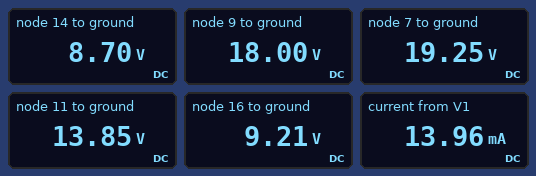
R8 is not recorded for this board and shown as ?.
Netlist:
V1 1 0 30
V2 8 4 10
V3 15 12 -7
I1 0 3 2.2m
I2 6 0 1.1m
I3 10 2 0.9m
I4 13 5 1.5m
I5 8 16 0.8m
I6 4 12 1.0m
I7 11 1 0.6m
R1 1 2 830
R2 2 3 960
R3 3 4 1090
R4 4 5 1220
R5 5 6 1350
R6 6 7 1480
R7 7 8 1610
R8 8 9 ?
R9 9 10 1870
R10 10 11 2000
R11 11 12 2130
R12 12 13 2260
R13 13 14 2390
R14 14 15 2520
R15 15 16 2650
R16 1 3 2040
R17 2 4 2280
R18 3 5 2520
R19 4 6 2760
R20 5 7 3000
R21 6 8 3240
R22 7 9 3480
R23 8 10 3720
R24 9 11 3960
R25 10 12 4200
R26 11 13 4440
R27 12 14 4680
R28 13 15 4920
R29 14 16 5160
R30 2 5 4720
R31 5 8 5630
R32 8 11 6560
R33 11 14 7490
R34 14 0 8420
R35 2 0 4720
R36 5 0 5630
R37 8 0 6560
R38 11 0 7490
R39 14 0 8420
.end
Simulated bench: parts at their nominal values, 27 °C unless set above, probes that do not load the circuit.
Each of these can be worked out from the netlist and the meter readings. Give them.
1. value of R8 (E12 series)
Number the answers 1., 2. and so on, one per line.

1. 3.3 kΩ
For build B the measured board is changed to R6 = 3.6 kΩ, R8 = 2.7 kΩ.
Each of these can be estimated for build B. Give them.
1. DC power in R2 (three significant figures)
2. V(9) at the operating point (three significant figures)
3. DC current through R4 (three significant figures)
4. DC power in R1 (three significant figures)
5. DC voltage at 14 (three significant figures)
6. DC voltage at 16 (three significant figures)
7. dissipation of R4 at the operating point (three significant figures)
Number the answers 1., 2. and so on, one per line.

1. 1.76 mW
2. 18.4 V
3. 3.12 mA
4. 81.7 mW
5. 8.85 V
6. 9.38 V
7. 11.9 mW
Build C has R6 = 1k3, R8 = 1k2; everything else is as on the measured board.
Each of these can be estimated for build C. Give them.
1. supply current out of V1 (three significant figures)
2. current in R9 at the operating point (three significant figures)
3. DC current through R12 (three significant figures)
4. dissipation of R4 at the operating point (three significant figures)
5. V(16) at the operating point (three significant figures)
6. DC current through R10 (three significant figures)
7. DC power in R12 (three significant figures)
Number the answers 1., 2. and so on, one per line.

1. 14.1 mA
2. 1.28 mA
3. 1.86 mA
4. 13.0 mW
5. 9.82 V
6. 1.35 mA
7. 7.83 mW
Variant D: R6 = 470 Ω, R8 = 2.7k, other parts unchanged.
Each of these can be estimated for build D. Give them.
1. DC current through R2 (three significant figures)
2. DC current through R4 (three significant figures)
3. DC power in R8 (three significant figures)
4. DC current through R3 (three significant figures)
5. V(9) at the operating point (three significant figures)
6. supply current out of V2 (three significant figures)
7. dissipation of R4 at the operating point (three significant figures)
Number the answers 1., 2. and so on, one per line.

1. 1.35 mA
2. 3.22 mA
3. 8.82 mW
4. 6.82 mA
5. 18.2 V
6. 14.6 mA
7. 12.7 mW
